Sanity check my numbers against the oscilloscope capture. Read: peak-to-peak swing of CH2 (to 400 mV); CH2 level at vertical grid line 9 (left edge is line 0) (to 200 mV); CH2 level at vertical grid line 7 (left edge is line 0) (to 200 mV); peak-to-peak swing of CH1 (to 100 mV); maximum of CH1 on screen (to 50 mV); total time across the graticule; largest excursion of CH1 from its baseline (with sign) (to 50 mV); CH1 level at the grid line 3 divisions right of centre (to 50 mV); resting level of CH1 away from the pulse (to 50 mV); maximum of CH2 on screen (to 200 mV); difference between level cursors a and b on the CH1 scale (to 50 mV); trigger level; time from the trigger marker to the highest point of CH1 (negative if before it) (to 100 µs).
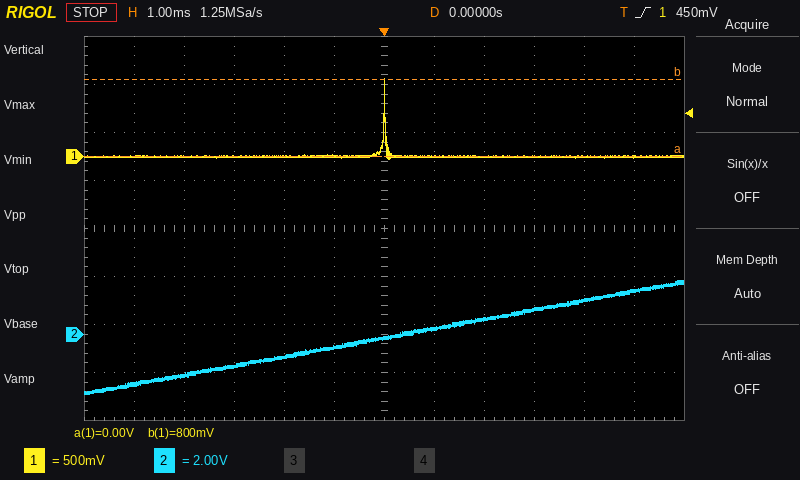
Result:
4.8 V
1.0 V
200 mV
800 mV
800 mV
12 ms
+800 mV
0 mV
0 mV
2.2 V
800 mV
450 mV
0.0 ms
